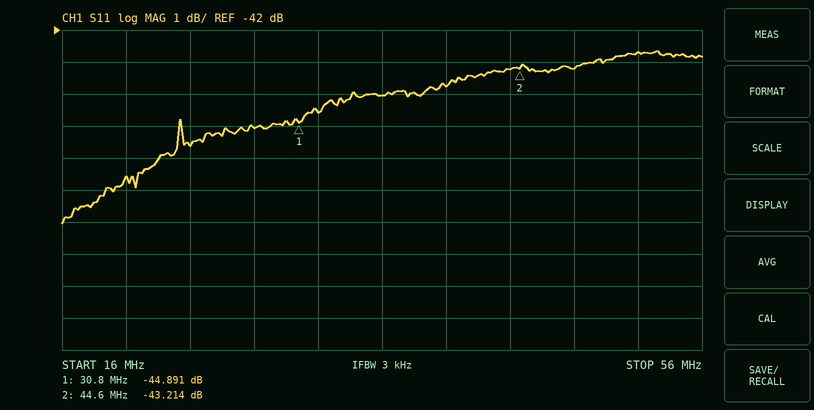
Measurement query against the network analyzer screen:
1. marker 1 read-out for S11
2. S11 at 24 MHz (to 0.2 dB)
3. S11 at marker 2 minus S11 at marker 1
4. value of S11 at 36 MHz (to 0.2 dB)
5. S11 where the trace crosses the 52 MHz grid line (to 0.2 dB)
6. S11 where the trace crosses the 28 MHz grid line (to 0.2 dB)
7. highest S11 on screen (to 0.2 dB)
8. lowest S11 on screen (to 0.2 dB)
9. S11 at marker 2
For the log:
-44.891 dB
-45.6 dB
1.677 dB
-44.0 dB
-42.6 dB
-45.0 dB
-42.6 dB
-48.0 dB
-43.214 dB
